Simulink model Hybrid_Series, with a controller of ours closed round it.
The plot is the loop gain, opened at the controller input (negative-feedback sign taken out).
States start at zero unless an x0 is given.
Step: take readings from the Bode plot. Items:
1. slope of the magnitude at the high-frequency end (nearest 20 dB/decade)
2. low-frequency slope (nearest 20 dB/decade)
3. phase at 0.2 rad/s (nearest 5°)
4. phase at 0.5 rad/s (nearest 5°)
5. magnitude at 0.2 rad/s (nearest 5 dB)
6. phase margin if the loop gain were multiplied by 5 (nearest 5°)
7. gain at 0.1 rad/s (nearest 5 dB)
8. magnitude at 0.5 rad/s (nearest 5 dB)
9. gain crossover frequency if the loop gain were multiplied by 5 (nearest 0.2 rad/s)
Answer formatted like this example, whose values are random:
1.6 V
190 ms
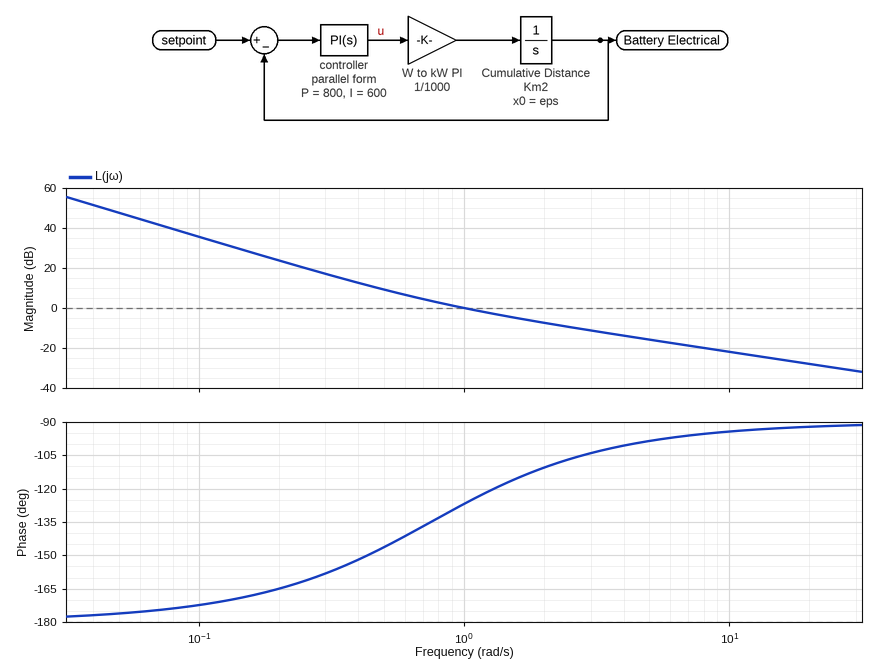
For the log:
-20 dB/decade
-40 dB/decade
-165°
-145°
25 dB
80°
35 dB
10 dB
4.0 rad/s
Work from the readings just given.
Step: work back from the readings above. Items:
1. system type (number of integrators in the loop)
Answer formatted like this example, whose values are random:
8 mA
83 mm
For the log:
2
